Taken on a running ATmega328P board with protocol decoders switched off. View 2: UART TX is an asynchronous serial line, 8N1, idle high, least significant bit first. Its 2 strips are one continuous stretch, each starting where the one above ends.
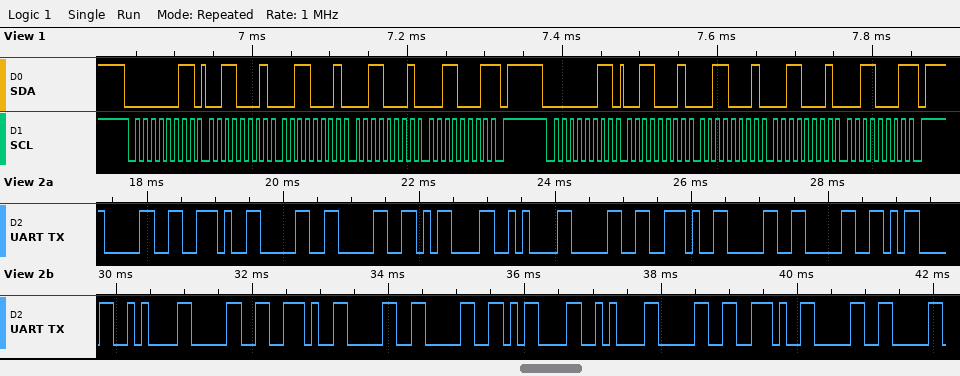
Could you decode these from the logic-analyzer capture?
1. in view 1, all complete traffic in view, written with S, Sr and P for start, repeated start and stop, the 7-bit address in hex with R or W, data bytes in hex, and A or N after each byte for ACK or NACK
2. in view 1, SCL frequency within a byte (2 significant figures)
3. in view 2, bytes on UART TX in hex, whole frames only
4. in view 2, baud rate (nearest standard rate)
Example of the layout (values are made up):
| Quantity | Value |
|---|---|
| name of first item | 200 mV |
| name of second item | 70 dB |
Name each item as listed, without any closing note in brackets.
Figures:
| Quantity | Value |
|---|---|
| in view 1, all complete traffic in view, written with S, Sr and P for start, repeated start and stop, the 7-bit address in hex with R or W, data bytes in hex, and A or N after each byte for ACK or NACK | S 01R A 31 A 31 A 31 A 31 N P S 01R A 31 A 31 A 31 A 31 N P |
| in view 1, SCL frequency within a byte | 100 kHz |
| in view 2, bytes on UART TX in hex, whole frames only | 0x30 0x2E 0x30 0x30 0x0D 0x0A 0x30 0x2E 0x30 0x30 0x0D 0x0A 0x30 0x2E 0x30 0x30 0x0D 0x0A 0x30 0x2E 0x30 |
| in view 2, baud rate | 9600 baud |
